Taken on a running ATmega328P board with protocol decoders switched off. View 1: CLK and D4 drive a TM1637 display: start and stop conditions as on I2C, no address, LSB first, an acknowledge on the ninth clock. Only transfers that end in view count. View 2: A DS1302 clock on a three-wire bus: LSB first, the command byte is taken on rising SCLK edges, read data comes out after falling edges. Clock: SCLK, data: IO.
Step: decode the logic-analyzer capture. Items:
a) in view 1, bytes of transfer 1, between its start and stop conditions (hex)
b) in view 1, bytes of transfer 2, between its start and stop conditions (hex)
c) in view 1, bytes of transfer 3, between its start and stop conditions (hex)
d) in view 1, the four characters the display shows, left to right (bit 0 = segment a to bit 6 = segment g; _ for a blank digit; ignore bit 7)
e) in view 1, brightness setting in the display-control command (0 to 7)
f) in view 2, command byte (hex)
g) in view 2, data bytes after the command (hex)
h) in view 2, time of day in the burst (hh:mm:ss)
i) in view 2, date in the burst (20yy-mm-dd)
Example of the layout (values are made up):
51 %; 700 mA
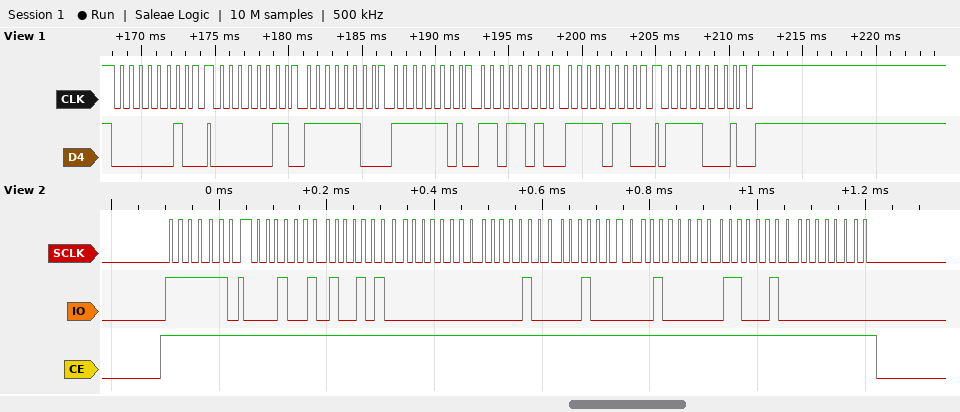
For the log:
40; C0 3F BF 5B 6F; 8F; 0029; 7; 0xBF; 48 29 00 10 04 02 23 00; 00:29:48; 2023-04-10
